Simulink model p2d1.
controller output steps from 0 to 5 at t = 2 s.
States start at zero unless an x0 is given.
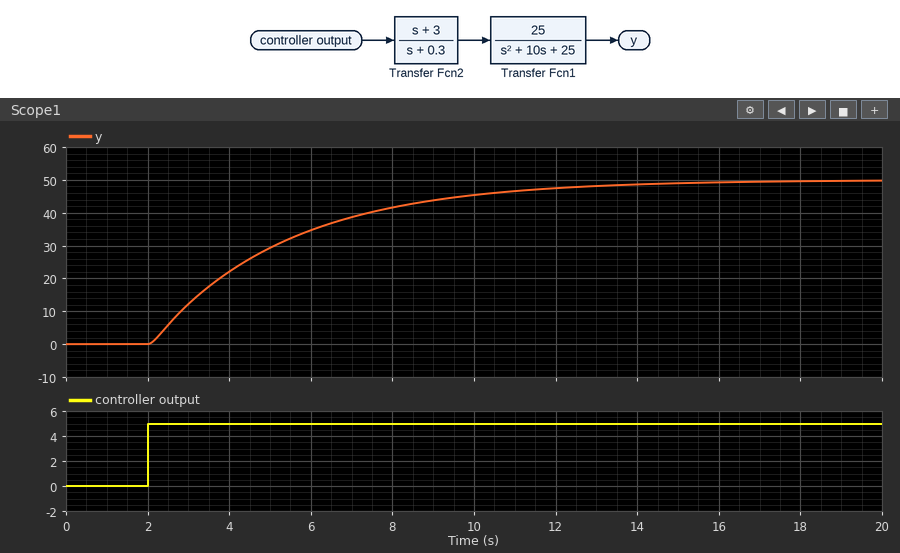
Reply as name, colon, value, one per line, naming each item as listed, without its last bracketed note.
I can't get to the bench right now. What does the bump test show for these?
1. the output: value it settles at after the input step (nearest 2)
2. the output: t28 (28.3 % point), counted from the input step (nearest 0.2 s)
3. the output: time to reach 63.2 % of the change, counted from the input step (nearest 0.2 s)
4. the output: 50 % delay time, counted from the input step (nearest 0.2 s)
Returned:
the output: value it settles at after the input step: 50
the output: t28 (28.3 % point), counted from the input step: 1.2 s
the output: time to reach 63.2 % of the change, counted from the input step: 3.4 s
the output: 50 % delay time, counted from the input step: 2.4 s
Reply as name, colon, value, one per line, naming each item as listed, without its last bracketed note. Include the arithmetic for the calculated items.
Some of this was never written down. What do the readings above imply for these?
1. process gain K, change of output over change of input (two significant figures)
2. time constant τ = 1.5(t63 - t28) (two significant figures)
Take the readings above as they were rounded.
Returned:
process gain K, change of output over change of input: (50 - 0) / 5 = 10
time constant τ = 1.5(t63 - t28): 1.5 × (3.4 - 1.2) = 3.3 s
